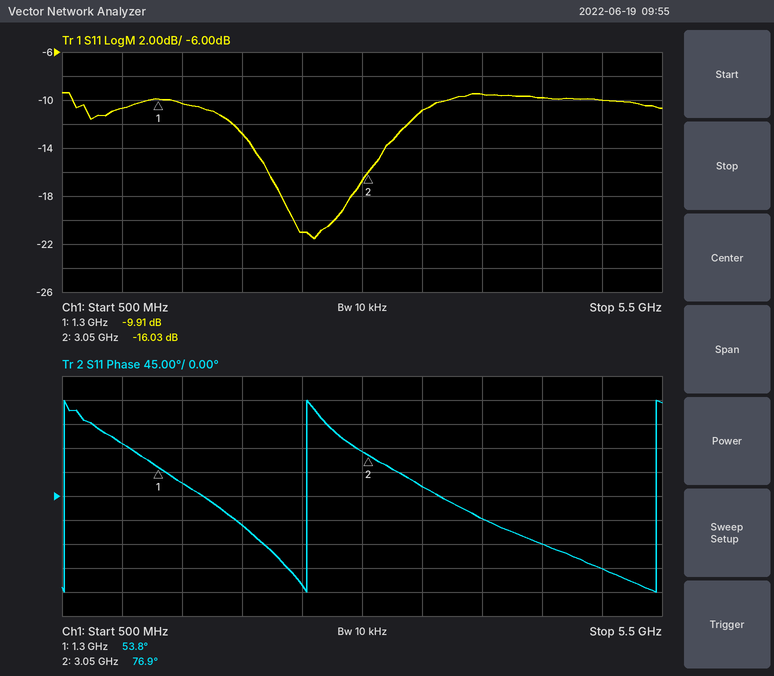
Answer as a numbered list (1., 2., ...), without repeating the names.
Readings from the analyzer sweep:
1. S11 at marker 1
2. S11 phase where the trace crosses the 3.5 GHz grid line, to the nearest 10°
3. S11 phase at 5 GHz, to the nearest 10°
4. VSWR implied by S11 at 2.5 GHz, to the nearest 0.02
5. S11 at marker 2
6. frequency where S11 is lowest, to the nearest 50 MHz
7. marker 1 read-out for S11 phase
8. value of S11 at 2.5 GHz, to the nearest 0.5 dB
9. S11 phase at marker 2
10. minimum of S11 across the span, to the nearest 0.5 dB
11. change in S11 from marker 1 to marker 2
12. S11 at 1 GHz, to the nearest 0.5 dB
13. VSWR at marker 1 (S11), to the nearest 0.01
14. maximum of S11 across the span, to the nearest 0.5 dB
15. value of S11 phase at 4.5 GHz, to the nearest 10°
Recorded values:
1. -9.91 dB
2. 20°
3. -140°
4. 1.20
5. -16.03 dB
6. 2.60 GHz
7. 53.8°
8. -21.0 dB
9. 76.9°
10. -21.5 dB
11. -6.12 dB
12. -10.5 dB
13. 1.94
14. -9.5 dB
15. -90°
